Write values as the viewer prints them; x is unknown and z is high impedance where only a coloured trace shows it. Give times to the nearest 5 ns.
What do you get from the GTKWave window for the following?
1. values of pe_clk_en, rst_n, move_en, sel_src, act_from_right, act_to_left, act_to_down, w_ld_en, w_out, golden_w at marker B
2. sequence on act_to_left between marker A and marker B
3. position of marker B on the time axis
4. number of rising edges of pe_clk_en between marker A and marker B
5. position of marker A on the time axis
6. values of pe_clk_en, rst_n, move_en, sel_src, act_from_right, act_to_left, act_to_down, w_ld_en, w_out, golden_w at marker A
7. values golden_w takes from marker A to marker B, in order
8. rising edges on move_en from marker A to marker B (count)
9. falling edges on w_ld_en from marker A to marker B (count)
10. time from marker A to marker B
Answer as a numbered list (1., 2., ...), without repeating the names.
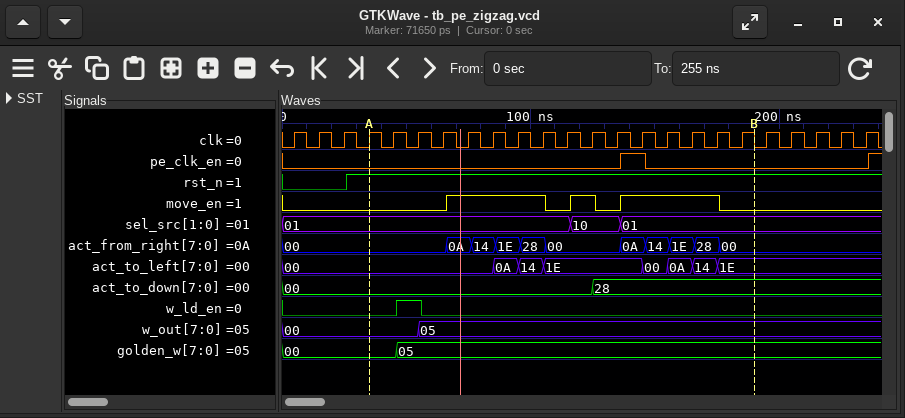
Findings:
1. pe_clk_en=0, rst_n=1, move_en=0, sel_src=01, act_from_right=00, act_to_left=1E, act_to_down=28, w_ld_en=0, w_out=05, golden_w=05
2. 00, 0A, 14, 1E, 00, 0A, 14, 1E
3. 190 ns
4. 1
5. 35 ns
6. pe_clk_en=0, rst_n=1, move_en=0, sel_src=01, act_from_right=00, act_to_left=00, act_to_down=00, w_ld_en=0, w_out=00, golden_w=00
7. 00, 05
8. 3
9. 1
10. 155 ns
